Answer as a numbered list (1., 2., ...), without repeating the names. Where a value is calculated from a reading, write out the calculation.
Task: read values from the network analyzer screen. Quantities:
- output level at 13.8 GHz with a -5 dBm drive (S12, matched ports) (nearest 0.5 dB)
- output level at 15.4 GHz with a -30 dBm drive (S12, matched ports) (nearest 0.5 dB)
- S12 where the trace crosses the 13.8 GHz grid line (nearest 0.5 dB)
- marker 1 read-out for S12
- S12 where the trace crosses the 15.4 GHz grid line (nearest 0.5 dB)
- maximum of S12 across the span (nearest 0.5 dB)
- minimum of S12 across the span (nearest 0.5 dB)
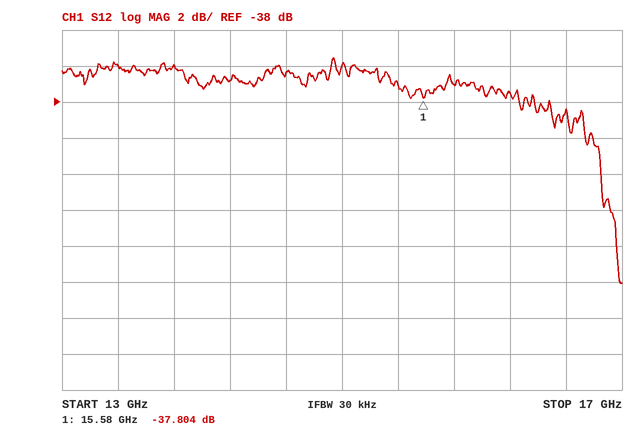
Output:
1. -5 dBm + (-36.0 dB) = -41.0 dBm
2. -30 dBm + (-37.0 dB) = -67.0 dBm
3. -36.0 dB
4. -37.804 dB
5. -37.0 dB
6. -35.5 dB
7. -48.0 dB
